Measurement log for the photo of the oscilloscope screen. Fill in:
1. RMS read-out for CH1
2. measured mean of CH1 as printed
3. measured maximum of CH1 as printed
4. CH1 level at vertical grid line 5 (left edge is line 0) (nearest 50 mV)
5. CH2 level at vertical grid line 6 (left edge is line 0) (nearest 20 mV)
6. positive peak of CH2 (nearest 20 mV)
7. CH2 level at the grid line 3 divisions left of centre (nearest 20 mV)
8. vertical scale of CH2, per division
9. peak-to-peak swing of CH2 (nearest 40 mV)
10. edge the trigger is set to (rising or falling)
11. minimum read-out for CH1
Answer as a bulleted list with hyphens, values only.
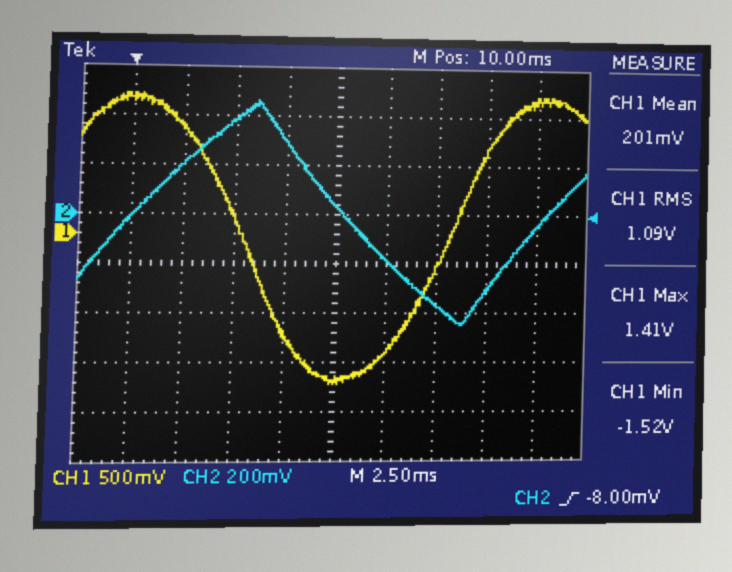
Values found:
- 1.09 V
- 201 mV
- 1.41 V
- -1.50 V
- -180 mV
- 460 mV
- 200 mV
- 200 mV
- 920 mV
- rising
- -1.52 V
